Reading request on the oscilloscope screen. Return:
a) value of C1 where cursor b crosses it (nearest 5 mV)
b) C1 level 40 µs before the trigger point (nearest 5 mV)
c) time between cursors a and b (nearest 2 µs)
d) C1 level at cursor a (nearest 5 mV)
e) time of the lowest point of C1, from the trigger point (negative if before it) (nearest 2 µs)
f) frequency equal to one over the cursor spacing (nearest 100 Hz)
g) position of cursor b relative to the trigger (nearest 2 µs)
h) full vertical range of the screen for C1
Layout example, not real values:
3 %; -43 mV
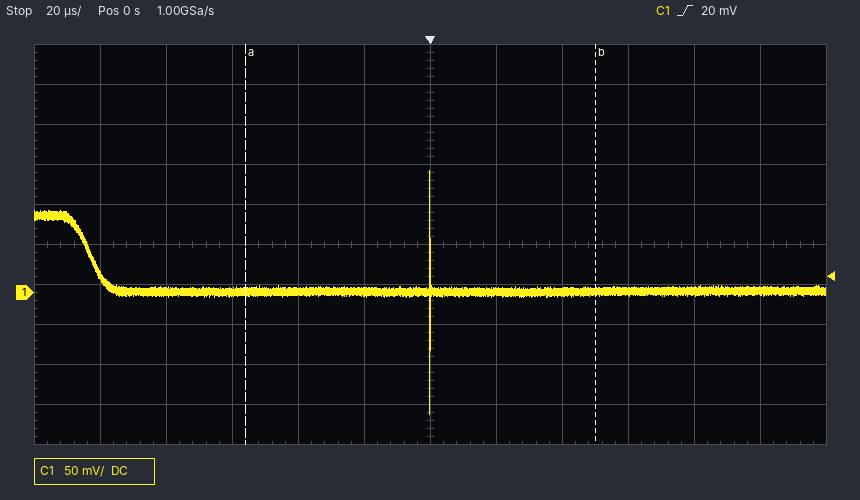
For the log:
0 mV; 0 mV; 106 µs; 0 mV; 0 µs; 9.4 kHz; +50 µs; 500 mV
